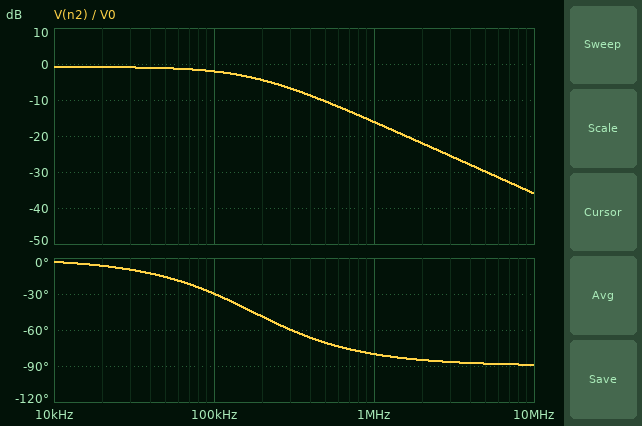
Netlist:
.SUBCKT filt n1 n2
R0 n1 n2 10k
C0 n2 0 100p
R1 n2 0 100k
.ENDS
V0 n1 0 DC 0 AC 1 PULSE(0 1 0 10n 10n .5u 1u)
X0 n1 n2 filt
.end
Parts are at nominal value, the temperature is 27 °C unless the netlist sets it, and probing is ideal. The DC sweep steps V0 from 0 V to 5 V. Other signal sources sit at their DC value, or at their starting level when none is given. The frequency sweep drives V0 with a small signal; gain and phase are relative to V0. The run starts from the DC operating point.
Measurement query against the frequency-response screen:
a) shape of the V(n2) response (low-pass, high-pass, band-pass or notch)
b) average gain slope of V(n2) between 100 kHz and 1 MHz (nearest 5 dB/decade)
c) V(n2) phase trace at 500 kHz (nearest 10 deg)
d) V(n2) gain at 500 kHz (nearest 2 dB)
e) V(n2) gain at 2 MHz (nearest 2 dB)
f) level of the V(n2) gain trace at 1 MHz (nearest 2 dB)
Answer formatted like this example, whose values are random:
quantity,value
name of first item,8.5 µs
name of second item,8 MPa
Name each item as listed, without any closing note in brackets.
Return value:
quantity,value
shape of the V(n2) response,low-pass
average gain slope of V(n2) between 100 kHz and 1 MHz,-15 dB/decade
V(n2) phase trace at 500 kHz,-70 deg
V(n2) gain at 500 kHz,-10 dB
V(n2) gain at 2 MHz,-22 dB
level of the V(n2) gain trace at 1 MHz,-16 dB
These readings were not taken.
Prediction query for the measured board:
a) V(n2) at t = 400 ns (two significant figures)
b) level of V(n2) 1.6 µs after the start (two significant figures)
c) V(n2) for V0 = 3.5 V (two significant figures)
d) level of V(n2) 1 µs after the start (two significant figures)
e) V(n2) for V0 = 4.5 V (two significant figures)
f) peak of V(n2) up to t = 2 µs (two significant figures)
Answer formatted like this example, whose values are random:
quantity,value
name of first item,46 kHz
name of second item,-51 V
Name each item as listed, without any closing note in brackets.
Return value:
quantity,value
V(n2) at t = 400 ns,320 mV
level of V(n2) 1.6 µs after the start,470 mV
V(n2) for V0 = 3.5 V,3.2 V
level of V(n2) 1 µs after the start,230 mV
V(n2) for V0 = 4.5 V,4.1 V
peak of V(n2) up to t = 2 µs,520 mV
